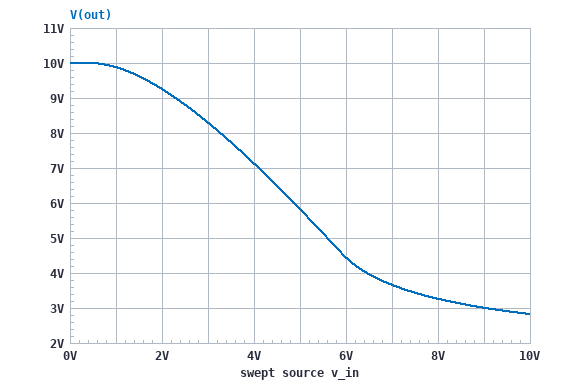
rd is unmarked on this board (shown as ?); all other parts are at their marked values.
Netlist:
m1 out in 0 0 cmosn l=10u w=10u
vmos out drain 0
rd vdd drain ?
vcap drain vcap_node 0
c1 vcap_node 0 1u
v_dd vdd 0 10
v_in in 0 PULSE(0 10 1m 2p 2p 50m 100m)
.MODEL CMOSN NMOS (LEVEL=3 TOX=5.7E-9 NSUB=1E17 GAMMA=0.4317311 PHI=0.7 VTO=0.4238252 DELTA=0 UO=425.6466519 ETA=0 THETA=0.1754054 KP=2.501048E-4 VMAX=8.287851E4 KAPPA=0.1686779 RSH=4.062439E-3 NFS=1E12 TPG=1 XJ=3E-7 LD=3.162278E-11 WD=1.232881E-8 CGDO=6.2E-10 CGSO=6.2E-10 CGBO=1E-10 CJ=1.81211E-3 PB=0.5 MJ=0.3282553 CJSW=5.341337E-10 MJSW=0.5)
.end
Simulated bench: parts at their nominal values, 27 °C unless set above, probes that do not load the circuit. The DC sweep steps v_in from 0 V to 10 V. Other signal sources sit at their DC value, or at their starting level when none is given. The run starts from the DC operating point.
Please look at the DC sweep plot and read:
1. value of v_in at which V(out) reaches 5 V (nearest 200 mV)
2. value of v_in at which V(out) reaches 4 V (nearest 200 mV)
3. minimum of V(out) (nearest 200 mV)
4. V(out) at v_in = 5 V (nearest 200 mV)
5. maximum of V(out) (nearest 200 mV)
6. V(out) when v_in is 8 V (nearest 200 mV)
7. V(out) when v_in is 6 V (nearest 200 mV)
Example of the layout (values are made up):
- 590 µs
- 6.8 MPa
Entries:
- 5.6 V
- 6.4 V
- 2.8 V
- 5.8 V
- 10.0 V
- 3.2 V
- 4.4 V
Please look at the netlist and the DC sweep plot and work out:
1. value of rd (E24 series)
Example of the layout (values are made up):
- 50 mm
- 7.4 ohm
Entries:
- 3.6 kΩ
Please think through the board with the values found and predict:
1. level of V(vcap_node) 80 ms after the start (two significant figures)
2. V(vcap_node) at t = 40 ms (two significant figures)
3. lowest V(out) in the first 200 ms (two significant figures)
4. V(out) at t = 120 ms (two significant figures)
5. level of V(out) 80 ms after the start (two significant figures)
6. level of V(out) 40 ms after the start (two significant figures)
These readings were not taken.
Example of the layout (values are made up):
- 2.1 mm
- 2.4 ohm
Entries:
- 10 V
- 2.8 V
- 2.8 V
- 2.8 V
- 10 V
- 2.8 V
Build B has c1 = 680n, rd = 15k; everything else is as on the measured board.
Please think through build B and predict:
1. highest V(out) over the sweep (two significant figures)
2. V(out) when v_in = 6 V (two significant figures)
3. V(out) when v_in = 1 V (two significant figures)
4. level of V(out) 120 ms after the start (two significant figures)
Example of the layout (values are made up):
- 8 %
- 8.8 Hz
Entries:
- 10 V
- 970 mV
- 9.5 V
- 730 mV
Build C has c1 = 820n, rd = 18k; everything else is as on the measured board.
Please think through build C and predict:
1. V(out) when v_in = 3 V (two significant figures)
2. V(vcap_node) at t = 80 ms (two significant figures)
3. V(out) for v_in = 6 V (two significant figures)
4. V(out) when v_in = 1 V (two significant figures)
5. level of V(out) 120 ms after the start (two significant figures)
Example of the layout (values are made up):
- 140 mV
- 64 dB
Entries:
- 1.8 V
- 8.7 V
- 810 mV
- 9.4 V
- 610 mV
